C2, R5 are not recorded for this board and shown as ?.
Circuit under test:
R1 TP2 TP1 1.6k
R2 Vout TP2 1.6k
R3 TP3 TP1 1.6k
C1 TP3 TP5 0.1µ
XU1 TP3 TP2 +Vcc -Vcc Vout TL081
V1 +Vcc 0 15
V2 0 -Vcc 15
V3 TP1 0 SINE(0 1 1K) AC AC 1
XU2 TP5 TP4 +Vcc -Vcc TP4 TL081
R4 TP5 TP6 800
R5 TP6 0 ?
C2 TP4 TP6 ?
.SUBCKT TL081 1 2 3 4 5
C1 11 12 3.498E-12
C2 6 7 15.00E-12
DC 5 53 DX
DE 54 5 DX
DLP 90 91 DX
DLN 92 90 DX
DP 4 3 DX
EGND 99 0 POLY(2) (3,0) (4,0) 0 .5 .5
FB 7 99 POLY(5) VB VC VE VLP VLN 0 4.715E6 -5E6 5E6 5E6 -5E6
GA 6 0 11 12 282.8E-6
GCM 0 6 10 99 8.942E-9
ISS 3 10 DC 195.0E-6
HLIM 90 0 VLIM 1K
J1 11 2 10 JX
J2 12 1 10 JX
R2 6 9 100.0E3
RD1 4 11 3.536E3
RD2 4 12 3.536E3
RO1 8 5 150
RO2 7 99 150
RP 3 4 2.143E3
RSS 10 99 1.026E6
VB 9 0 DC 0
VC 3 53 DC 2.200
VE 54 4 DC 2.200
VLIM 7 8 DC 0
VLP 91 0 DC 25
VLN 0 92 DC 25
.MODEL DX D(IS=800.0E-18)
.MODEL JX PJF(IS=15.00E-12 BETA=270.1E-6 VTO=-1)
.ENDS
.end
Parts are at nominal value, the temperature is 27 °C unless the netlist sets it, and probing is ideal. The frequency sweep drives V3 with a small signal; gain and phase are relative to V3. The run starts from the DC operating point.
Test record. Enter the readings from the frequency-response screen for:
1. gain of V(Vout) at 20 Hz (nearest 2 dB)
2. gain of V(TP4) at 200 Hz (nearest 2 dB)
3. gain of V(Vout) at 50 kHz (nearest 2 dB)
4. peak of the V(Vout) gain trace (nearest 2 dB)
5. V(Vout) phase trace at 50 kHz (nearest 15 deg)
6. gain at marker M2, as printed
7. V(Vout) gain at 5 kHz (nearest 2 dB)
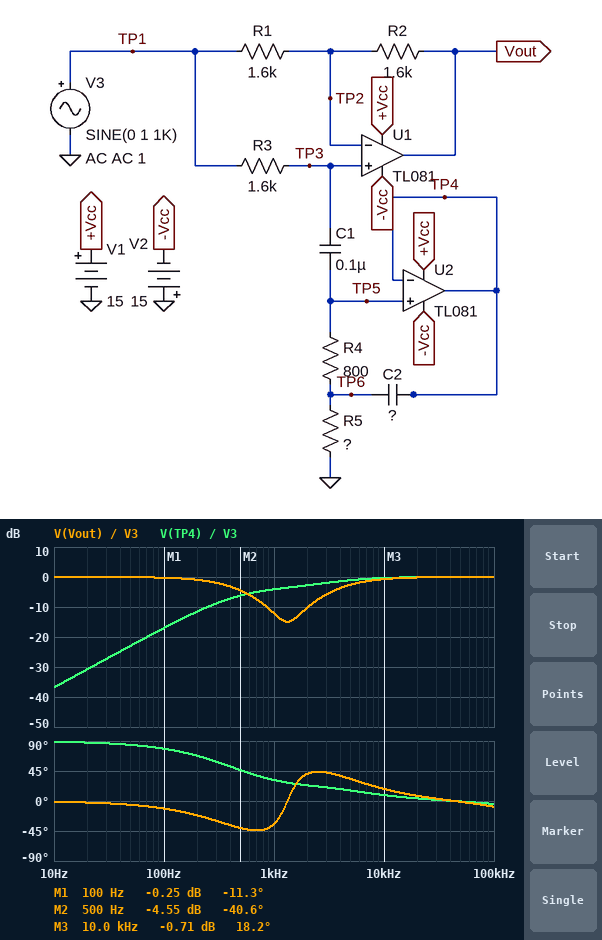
0 dB
-12 dB
0 dB
0 dB
0 deg
-4.55 dB
-2 dB
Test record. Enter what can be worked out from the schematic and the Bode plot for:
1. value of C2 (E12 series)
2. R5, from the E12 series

120 nF
1.5 kΩ
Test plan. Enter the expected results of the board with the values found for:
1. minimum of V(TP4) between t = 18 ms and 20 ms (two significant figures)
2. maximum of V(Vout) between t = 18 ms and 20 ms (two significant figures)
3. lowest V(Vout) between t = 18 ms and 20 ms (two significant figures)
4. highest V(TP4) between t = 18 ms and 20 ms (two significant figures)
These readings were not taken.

-620 mV
250 mV
-250 mV
620 mV
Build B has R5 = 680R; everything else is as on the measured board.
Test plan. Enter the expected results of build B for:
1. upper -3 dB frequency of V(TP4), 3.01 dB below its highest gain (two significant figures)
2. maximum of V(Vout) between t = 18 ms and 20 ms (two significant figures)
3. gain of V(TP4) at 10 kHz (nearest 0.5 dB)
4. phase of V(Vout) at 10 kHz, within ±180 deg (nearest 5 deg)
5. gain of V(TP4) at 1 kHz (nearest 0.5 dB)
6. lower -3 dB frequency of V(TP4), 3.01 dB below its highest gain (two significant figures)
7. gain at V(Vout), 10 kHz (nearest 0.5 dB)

1.0 MHz
360 mV
-1.0 dB
40 deg
-6.5 dB
4.8 kHz
-2.0 dB
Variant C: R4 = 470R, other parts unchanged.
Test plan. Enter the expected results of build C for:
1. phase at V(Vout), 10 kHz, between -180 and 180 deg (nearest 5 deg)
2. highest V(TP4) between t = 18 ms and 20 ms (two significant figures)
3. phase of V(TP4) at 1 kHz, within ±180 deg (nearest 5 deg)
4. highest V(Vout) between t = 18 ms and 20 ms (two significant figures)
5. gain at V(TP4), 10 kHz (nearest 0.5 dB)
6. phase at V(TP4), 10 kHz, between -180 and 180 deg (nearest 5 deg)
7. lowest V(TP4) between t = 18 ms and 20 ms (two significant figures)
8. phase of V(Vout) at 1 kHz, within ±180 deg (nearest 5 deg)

30 deg
550 mV
30 deg
300 mV
-1.0 dB
15 deg
-550 mV
-55 deg
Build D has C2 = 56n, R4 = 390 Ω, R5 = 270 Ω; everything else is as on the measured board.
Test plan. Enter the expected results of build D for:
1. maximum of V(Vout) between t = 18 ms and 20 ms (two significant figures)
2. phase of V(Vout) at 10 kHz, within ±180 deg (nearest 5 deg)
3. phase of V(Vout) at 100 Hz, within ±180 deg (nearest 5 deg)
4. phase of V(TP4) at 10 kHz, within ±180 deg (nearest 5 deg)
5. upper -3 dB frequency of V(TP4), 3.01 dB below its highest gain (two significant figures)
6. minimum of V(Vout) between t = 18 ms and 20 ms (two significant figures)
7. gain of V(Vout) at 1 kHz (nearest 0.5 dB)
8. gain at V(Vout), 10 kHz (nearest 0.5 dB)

660 mV
160 deg
-10 deg
25 deg
490 kHz
-660 mV
-3.5 dB
-7.5 dB
